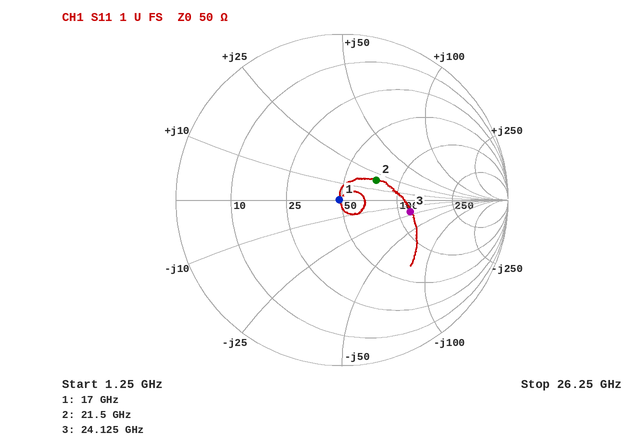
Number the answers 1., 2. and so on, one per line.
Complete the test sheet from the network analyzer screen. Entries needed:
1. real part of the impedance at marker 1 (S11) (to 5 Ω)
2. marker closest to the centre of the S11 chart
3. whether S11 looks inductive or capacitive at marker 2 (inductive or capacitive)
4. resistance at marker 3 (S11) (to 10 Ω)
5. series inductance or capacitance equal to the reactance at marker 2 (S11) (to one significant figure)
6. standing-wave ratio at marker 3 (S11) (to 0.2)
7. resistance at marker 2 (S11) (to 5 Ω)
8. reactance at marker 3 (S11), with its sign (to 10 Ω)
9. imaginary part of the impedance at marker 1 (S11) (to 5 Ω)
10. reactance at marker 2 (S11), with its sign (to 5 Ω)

1. 50 Ω
2. marker 1
3. inductive
4. 120 Ω
5. 100 pH
6. 2.4
7. 75 Ω
8. -20 Ω
9. 0 Ω
10. +20 Ω
